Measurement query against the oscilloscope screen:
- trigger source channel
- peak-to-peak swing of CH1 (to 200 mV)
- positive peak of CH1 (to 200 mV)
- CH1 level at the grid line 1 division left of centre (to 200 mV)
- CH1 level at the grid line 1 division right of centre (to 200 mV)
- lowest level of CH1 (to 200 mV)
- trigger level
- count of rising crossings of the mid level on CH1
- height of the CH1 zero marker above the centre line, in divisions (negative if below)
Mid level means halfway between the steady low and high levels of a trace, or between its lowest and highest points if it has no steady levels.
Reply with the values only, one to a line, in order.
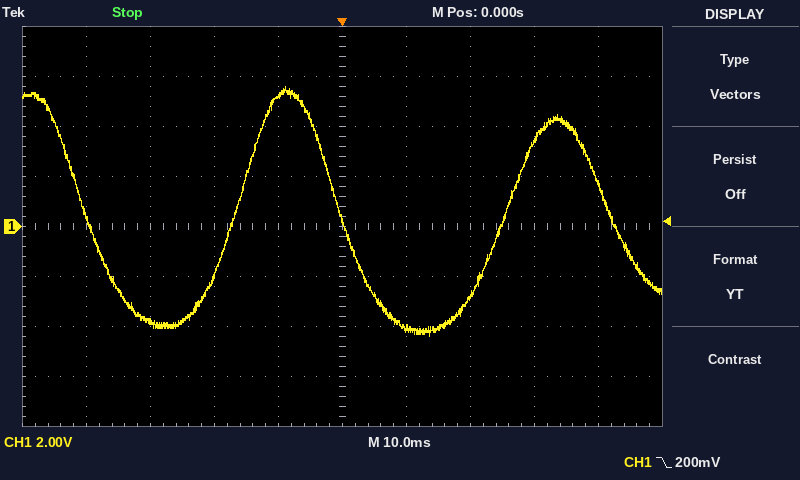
CH1
10.0 V
5.6 V
5.2 V
-4.0 V
-4.4 V
200 mV
2
0.0 div
